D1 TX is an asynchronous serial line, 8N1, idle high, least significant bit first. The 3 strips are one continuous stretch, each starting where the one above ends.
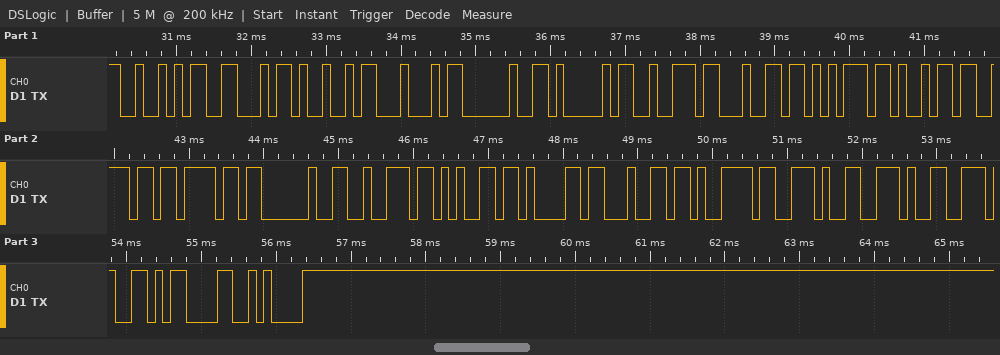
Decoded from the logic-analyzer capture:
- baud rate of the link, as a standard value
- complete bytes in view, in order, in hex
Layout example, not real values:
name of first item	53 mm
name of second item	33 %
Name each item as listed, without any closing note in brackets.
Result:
baud rate of the link, as a standard value	9600 baud
complete bytes in view, in order, in hex	52 46 49 44 20 41 72 64 75 69 6E 6F 20 72 65 61 64 79 2E 2E 2E 0D 0A
